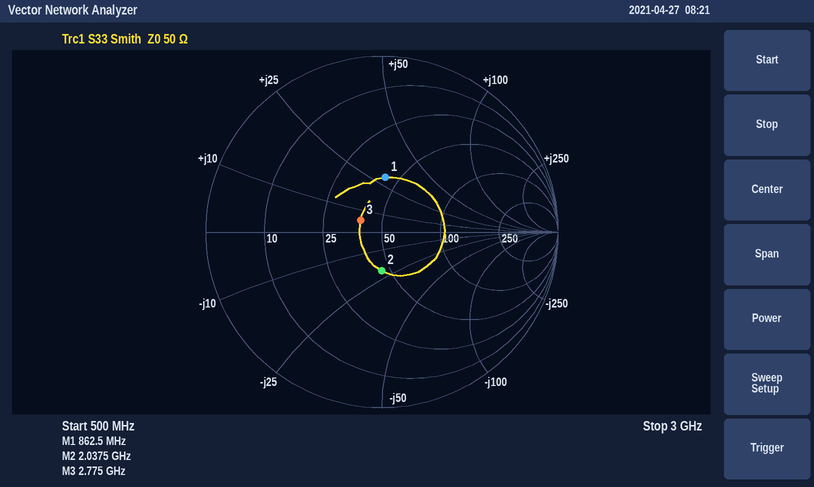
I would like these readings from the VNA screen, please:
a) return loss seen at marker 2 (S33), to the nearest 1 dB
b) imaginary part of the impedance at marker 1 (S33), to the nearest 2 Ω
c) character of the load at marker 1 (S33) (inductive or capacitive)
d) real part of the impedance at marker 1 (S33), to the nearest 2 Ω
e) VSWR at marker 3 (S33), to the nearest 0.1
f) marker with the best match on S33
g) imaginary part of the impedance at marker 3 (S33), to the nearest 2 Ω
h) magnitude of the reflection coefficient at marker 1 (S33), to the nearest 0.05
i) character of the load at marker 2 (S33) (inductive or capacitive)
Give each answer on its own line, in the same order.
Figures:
13 dB
+30 Ω
inductive
42 Ω
1.3
marker 3
+6 Ω
0.30
capacitive
